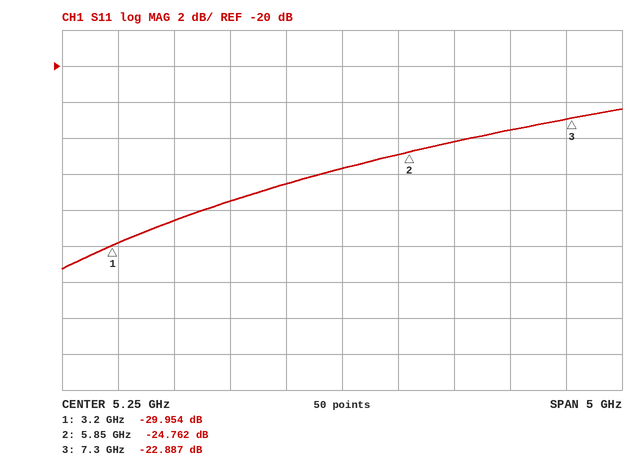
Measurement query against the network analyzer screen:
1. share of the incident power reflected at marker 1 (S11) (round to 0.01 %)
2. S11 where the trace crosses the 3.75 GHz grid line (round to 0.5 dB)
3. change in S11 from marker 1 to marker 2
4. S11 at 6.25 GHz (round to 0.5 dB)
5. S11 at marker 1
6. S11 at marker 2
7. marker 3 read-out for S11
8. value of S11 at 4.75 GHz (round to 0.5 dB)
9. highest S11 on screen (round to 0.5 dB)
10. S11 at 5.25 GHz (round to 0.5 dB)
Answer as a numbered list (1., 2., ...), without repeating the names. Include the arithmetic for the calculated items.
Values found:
1. 10^(-29.954/10) ≈ 0.10 %
2. -28.5 dB
3. -24.762 − (-29.954) = 5.192 dB
4. -24.0 dB
5. -29.954 dB
6. -24.762 dB
7. -22.887 dB
8. -26.5 dB
9. -22.5 dB
10. -25.5 dB
